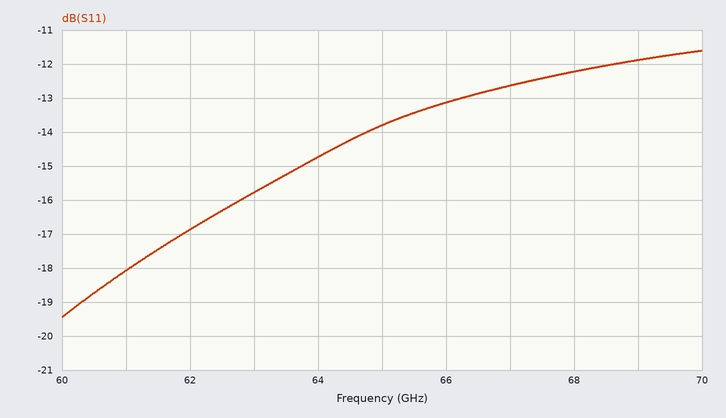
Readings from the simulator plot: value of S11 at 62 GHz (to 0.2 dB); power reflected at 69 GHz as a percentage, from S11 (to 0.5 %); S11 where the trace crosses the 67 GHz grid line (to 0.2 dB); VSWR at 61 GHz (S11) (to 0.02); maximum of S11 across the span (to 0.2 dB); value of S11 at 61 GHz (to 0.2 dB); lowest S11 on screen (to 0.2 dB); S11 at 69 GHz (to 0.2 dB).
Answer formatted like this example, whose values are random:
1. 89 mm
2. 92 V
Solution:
1. -16.8 dB
2. 6.5 %
3. -12.6 dB
4. 1.28
5. -11.6 dB
6. -18.0 dB
7. -19.4 dB
8. -11.8 dB
